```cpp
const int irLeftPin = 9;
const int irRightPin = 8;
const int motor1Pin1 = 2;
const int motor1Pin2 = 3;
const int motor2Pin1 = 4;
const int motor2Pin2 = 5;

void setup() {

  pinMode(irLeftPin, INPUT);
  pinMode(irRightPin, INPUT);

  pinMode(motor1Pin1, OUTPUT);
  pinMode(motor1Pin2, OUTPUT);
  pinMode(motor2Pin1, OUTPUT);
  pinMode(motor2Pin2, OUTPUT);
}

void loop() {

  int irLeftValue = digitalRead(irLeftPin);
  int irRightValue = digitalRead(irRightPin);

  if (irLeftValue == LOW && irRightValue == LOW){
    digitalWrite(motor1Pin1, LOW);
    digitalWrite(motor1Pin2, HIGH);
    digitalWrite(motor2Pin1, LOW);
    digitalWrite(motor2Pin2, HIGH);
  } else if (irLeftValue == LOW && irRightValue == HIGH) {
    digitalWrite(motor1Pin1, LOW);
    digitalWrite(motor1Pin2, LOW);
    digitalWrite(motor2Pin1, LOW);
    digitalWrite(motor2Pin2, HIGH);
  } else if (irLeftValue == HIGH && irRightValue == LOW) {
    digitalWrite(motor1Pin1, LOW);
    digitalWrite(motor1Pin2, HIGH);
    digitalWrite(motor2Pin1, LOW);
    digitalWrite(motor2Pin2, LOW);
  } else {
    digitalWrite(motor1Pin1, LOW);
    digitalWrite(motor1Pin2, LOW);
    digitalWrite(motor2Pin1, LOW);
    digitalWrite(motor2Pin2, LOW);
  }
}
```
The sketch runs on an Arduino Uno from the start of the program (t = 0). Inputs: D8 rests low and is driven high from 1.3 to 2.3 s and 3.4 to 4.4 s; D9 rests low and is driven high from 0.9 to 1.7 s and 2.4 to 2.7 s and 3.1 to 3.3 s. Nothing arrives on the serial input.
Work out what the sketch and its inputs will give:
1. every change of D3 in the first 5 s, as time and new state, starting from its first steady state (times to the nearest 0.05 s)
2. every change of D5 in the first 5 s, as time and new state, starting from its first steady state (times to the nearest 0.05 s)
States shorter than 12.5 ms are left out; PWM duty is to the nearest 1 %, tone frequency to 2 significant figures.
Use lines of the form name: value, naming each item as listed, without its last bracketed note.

every change of D3 in the first 5 s, as time and new state, starting from its first steady state: 0 s high; 1.3 s low; 2.3 s high; 3.4 s low; 4.4 s high
every change of D5 in the first 5 s, as time and new state, starting from its first steady state: 0 s high; 0.9 s low; 1.7 s high; 2.4 s low; 2.7 s high; 3.1 s low; 3.3 s high
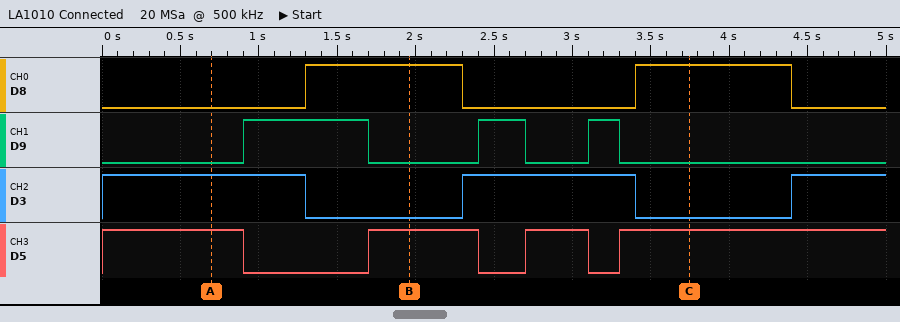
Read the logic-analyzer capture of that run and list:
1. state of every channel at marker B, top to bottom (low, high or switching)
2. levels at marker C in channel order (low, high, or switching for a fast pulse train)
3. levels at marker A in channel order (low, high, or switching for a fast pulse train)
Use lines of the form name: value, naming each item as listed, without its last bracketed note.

state of every channel at marker B, top to bottom: D8 high, D9 low, D3 low, D5 high
levels at marker C in channel order: D8 high, D9 low, D3 low, D5 high
levels at marker A in channel order: D8 low, D9 low, D3 high, D5 high
